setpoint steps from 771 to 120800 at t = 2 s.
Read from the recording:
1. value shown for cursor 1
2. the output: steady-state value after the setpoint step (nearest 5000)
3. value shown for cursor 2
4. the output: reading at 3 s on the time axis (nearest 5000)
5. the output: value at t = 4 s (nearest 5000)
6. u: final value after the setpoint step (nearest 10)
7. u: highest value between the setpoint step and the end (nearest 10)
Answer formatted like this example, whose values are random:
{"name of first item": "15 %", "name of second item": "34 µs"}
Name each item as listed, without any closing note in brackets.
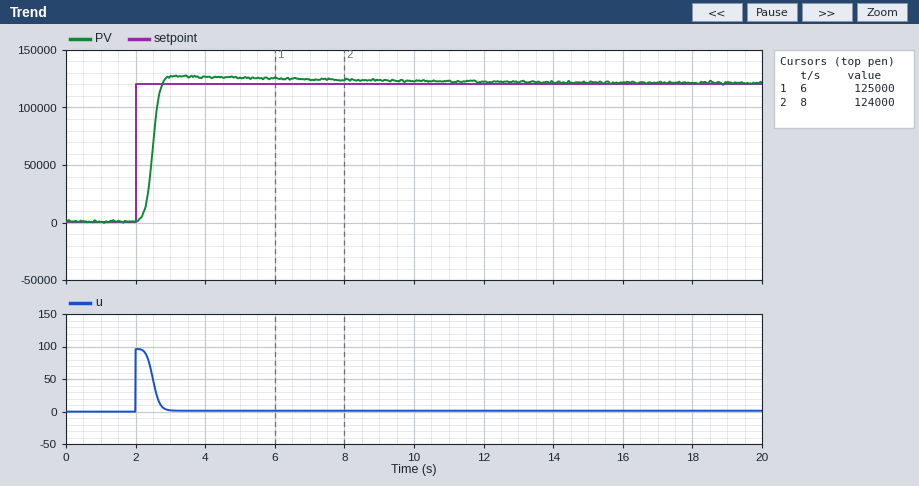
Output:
{"value shown for cursor 1": "125000", "the output: steady-state value after the setpoint step": "120000", "value shown for cursor 2": "124000", "the output: reading at 3 s on the time axis": "125000", "the output: value at t = 4 s": "125000", "u: final value after the setpoint step": "0", "u: highest value between the setpoint step and the end": "100"}
